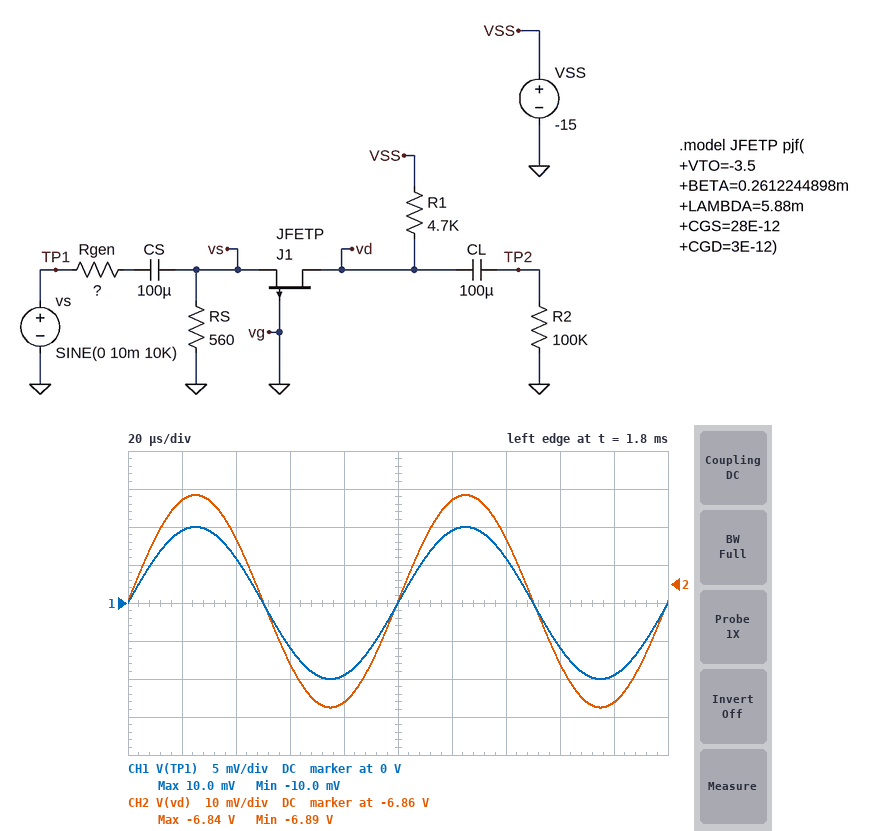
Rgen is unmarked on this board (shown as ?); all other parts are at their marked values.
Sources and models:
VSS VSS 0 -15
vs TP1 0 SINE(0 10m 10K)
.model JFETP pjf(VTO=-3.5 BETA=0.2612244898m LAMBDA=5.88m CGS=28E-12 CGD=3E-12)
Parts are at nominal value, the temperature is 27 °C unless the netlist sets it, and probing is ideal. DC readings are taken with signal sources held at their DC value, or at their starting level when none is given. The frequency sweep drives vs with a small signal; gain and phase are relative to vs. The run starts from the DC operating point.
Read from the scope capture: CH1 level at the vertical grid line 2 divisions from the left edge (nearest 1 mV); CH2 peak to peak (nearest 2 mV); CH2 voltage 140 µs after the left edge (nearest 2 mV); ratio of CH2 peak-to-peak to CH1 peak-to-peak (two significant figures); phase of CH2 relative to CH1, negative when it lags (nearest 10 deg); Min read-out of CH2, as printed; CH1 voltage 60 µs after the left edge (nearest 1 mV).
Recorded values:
6 mV
56 mV
-6.848 V
2.8
0 deg
-6.89 V
-6 mV
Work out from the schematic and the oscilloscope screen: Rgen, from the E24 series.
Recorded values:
360 Ω
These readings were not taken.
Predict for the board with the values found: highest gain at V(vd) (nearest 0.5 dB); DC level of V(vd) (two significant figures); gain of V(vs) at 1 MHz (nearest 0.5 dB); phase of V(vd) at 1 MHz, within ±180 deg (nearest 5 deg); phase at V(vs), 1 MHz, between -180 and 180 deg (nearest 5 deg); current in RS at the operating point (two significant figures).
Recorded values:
9.0 dB
-6.9 V
-6.5 dB
-5 deg
0 deg
1.7 mA
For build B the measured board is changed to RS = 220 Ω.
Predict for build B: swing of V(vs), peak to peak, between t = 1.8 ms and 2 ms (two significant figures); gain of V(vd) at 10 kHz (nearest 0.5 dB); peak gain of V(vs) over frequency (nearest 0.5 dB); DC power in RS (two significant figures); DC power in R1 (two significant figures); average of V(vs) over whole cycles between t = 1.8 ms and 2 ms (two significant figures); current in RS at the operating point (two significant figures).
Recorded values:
6.3 mV
6.5 dB
-10.0 dB
1.2 mW
26 mW
-520 mV
2.4 mA
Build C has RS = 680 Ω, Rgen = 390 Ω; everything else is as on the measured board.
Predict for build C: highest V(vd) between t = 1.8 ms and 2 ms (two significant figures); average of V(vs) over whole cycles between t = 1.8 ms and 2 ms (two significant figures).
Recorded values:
-7.5 V
-1.1 V
